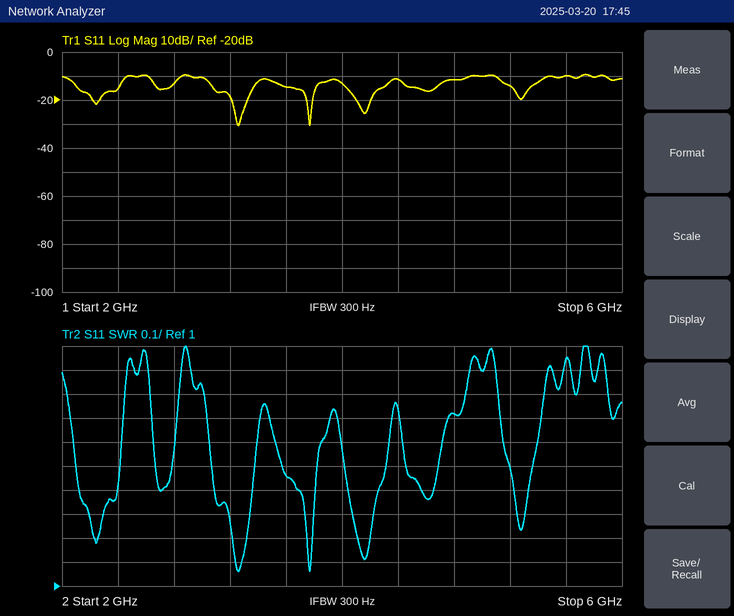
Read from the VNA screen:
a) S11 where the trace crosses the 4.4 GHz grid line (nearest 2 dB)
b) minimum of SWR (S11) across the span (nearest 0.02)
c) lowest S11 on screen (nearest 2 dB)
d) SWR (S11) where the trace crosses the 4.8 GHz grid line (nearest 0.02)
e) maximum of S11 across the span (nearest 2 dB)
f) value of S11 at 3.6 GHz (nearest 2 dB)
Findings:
-12 dB
1.06
-30 dB
1.72
-10 dB
-14 dB
